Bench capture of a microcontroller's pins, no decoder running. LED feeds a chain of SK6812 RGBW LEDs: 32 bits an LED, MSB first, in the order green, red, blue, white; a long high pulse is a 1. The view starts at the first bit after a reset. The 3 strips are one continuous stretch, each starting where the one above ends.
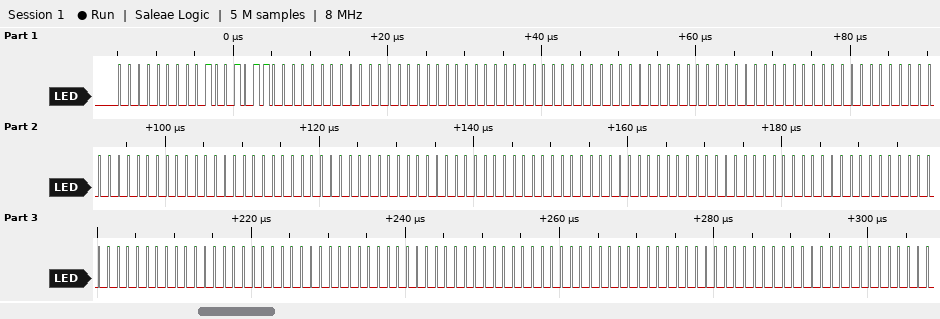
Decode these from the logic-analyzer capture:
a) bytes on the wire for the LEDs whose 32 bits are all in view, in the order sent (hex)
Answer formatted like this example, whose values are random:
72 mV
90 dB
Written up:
00 4B 00 00 00 00 00 00 00 00 00 00 00 00 00 00 00 00 00 00 00 00 00 00 00 00 00 00 00 00 00 00
